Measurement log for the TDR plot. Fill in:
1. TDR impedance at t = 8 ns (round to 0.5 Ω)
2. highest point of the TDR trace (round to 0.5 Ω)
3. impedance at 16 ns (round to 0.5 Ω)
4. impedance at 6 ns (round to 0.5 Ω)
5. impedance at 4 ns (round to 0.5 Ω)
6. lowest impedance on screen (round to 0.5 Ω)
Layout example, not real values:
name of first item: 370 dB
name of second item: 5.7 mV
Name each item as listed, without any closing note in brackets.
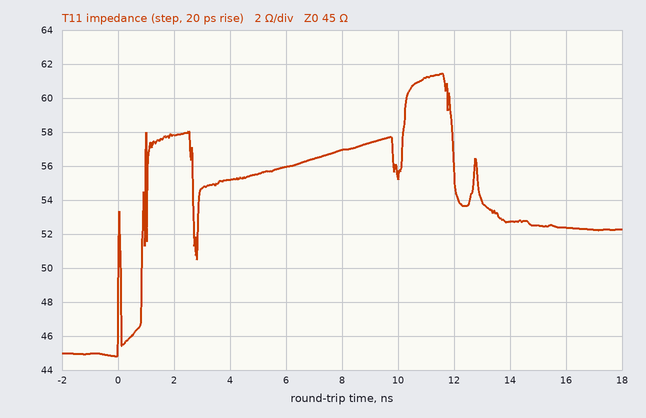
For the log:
TDR impedance at t = 8 ns: 57.0 Ω
highest point of the TDR trace: 61.5 Ω
impedance at 16 ns: 52.5 Ω
impedance at 6 ns: 56.0 Ω
impedance at 4 ns: 55.0 Ω
lowest impedance on screen: 45.0 Ω
